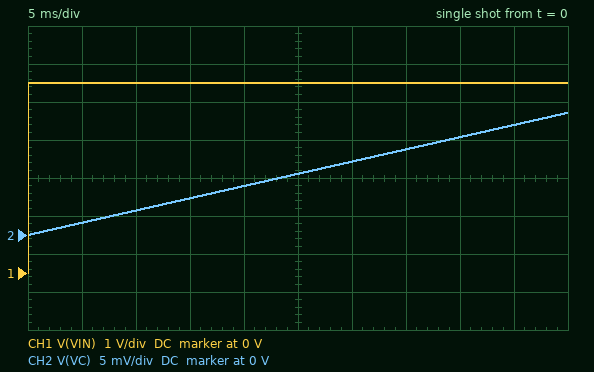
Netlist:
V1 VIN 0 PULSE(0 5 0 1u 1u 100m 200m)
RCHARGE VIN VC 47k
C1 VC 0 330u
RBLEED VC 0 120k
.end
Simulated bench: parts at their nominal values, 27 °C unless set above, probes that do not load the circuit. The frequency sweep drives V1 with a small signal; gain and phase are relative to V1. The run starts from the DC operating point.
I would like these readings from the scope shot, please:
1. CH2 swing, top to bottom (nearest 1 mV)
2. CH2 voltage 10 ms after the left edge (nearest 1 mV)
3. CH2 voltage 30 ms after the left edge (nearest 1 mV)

16 mV
3 mV
10 mV
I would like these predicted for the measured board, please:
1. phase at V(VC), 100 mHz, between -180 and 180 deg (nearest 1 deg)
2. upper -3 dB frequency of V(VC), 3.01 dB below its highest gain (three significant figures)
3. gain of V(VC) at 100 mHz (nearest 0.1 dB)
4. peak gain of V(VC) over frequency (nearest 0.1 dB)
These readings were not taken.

-82 deg
14.3 mHz
-19.9 dB
-2.9 dB
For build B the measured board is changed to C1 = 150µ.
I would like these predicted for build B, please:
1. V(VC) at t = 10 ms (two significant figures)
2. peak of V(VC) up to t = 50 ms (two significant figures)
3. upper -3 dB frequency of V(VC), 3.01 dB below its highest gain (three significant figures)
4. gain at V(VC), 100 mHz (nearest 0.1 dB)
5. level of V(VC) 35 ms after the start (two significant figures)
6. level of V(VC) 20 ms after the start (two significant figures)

7.1 mV
35 mV
31.4 mHz
-13.3 dB
25 mV
14 mV
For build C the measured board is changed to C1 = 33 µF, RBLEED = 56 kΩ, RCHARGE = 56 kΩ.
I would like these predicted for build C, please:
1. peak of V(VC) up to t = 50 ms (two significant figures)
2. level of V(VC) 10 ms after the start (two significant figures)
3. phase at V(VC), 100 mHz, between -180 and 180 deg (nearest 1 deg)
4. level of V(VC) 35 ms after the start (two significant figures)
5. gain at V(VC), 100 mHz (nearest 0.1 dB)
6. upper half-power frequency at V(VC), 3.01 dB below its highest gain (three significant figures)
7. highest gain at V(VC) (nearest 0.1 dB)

130 mV
27 mV
-30 deg
93 mV
-7.3 dB
172 mHz
-6.0 dB
